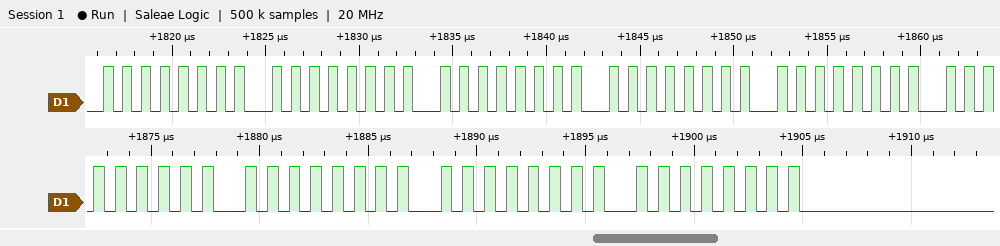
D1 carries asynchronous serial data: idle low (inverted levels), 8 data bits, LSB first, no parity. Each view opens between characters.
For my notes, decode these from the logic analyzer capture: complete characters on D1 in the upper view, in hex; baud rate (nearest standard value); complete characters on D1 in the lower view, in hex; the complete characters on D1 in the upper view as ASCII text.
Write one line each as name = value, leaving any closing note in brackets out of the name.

complete characters on D1 in the upper view, in hex = 55, 75, 55, 5D, 55, 57, 55, 55, 75
baud rate = 2000000 baud
complete characters on D1 in the lower view, in hex = 55, 57, 55, 55, 75, 55, FD
the complete characters on D1 in the upper view as ASCII text = "UuU]UWUUu"
